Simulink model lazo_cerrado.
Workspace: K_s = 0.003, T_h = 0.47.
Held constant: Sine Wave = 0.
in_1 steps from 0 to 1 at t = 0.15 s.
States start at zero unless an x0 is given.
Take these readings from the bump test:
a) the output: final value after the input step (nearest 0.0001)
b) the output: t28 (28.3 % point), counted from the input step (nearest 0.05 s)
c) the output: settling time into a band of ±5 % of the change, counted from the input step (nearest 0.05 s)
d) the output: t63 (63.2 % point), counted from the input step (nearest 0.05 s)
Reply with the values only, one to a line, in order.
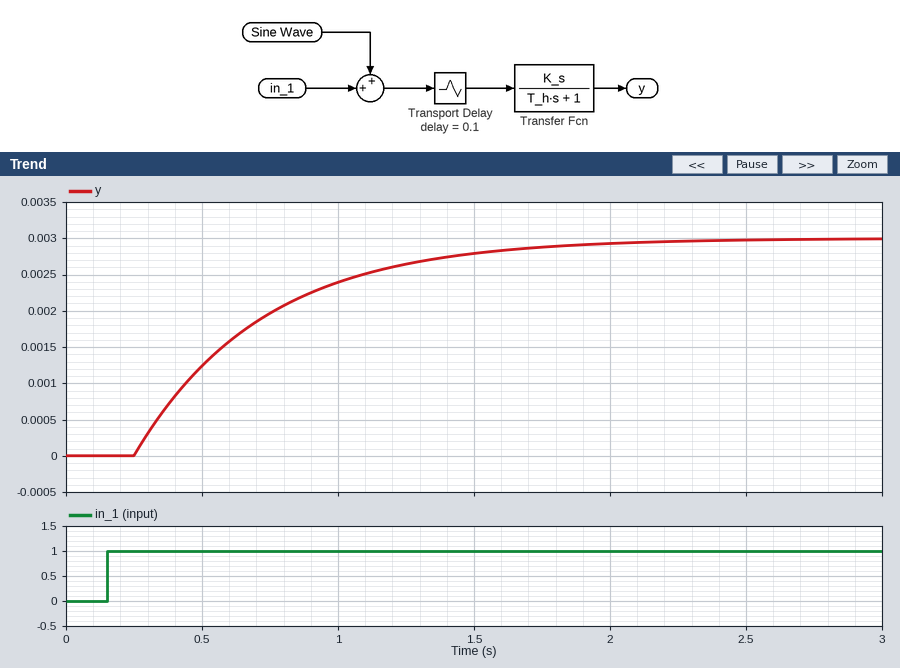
0.0030
0.25 s
1.50 s
0.55 s
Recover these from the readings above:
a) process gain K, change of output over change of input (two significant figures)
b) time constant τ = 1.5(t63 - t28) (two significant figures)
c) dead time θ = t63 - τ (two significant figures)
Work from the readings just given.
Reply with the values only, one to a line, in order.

0.0030
0.45 s
0.10 s
